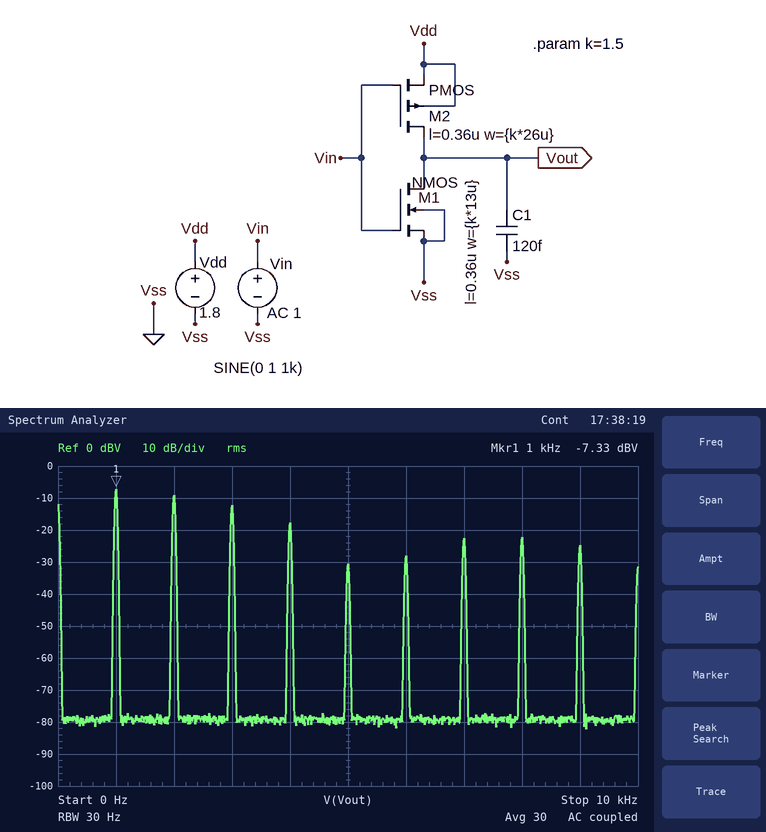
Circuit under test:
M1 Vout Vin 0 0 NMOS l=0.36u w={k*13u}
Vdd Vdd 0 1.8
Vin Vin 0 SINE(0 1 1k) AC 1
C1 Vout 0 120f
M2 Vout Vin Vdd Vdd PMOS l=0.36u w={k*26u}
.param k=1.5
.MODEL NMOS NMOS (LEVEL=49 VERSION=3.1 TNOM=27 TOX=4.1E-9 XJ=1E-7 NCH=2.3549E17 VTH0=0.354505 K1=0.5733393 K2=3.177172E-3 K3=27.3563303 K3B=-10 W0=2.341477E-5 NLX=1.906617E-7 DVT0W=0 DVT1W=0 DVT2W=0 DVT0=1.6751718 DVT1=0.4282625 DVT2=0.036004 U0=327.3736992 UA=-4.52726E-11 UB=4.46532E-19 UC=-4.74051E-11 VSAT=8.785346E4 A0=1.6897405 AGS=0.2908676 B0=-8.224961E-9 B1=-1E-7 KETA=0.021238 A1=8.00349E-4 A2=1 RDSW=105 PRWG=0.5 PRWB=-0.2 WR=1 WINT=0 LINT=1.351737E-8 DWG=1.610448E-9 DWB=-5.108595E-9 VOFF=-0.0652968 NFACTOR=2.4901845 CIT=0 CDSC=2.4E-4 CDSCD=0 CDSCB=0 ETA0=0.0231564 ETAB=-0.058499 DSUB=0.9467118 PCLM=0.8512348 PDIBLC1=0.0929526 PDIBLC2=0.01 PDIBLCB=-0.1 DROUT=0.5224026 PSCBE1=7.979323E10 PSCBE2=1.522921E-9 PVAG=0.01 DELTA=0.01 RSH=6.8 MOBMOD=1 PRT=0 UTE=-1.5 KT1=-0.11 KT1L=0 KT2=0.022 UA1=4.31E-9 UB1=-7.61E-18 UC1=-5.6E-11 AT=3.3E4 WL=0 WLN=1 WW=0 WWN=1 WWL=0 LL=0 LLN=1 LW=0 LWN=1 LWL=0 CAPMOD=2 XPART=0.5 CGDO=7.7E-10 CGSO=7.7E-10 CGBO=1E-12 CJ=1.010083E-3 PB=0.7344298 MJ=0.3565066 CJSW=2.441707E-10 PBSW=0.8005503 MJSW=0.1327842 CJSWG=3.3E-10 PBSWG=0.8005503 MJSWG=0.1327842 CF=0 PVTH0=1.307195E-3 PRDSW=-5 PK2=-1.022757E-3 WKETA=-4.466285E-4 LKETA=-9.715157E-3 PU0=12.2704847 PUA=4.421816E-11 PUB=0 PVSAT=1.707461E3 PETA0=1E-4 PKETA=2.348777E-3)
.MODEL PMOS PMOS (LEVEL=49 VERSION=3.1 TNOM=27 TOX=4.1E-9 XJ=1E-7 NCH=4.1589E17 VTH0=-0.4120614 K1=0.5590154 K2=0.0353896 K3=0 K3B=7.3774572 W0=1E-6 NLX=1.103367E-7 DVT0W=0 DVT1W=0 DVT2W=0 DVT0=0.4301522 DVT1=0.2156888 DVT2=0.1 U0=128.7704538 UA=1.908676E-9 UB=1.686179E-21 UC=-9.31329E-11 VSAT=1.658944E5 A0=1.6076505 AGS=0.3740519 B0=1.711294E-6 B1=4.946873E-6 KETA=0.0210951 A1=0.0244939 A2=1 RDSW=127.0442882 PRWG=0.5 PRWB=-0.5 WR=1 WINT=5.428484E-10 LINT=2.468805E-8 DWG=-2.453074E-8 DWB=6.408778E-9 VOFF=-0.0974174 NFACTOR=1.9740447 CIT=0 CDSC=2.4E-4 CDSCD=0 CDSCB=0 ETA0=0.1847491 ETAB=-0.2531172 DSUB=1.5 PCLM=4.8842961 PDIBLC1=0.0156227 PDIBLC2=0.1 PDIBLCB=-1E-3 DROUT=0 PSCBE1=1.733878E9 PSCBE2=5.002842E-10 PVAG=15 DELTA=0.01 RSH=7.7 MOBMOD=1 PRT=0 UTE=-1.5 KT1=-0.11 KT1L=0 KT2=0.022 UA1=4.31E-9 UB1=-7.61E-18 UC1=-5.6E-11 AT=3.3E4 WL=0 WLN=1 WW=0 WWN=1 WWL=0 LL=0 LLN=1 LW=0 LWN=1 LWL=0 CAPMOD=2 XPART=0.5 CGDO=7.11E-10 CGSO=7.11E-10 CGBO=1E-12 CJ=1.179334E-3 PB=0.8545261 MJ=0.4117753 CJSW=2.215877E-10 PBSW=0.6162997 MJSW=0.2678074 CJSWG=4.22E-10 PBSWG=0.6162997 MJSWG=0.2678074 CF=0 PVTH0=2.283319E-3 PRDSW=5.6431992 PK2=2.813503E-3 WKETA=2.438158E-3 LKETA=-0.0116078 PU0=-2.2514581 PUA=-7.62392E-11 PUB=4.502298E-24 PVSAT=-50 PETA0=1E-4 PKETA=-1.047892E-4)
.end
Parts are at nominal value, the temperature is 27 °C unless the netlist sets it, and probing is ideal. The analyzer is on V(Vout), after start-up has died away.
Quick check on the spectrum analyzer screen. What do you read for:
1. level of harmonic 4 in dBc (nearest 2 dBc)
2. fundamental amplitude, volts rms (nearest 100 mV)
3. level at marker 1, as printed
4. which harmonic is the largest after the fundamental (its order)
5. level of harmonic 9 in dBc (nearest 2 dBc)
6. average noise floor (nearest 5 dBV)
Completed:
-10 dBc
400 mV
-7.33 dBV
2
-18 dBc
-80 dBV
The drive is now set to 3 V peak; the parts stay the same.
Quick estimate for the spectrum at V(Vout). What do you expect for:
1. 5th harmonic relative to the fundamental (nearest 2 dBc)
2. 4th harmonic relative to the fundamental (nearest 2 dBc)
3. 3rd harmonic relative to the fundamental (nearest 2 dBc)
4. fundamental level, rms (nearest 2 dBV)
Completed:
-30 dBc
-12 dBc
-12 dBc
-2 dBV
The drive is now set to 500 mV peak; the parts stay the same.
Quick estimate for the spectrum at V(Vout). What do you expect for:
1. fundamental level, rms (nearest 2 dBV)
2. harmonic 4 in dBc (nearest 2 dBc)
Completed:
-66 dBV
-6 dBc
